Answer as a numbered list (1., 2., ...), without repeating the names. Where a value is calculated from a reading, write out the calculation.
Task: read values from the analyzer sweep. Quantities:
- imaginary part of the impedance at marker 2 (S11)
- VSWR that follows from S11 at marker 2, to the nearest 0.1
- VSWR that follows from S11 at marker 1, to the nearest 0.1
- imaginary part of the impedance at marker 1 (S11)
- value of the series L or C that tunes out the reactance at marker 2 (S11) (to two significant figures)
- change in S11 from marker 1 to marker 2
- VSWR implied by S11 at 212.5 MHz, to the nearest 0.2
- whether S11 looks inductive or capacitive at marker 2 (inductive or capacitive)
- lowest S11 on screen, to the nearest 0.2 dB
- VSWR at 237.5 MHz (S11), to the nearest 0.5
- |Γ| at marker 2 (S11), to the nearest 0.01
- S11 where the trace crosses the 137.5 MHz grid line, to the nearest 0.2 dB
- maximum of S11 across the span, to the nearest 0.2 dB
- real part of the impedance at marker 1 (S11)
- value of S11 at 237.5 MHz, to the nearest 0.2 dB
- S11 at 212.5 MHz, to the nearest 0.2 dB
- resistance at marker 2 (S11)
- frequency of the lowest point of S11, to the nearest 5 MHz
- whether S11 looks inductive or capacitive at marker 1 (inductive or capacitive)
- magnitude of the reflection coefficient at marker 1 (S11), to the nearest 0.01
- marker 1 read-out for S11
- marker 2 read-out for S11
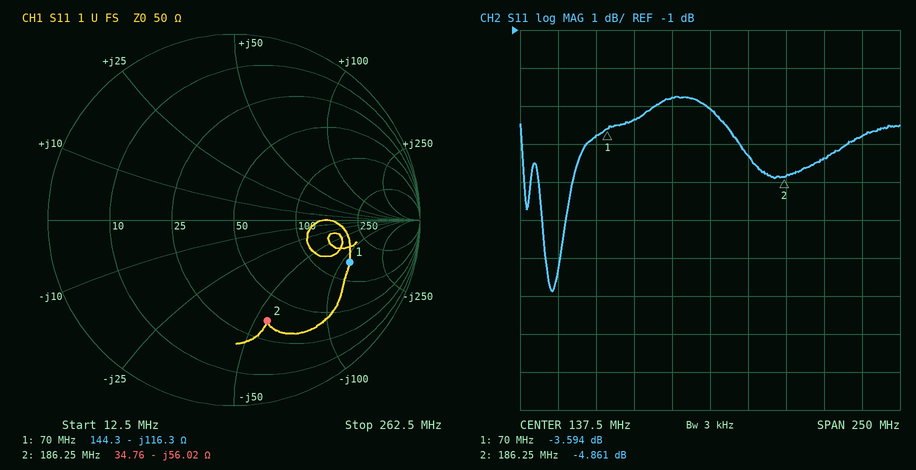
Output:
1. -56.02 Ω
2. (1 + 0.5714)/(1 − 0.5714) ≈ 3.7
3. (1 + 0.6611)/(1 − 0.6611) ≈ 4.9
4. -116.3 Ω
5. L = 56.02 Ω/(2π × 186.25 MHz) ≈ 48 nH
6. -4.861 − (-3.594) = -1.267 dB
7. |Γ| = 10^(-4.4/20) = 0.6026; VSWR = (1 + 0.6026)/(1 − 0.6026) ≈ 4.0
8. capacitive
9. -7.8 dB
10. |Γ| = 10^(-3.8/20) = 0.6457; VSWR = (1 + 0.6457)/(1 − 0.6457) ≈ 4.64, so 4.5 to the nearest 0.5
11. 0.57
12. -3.0 dB
13. -2.8 dB
14. 144.3 Ω
15. -3.8 dB
16. -4.4 dB
17. 34.76 Ω
18. 35 MHz
19. capacitive
20. 0.66
21. -3.594 dB
22. -4.861 dB
